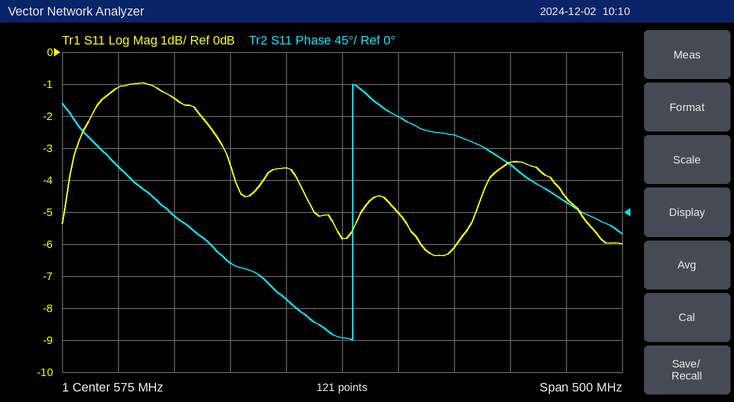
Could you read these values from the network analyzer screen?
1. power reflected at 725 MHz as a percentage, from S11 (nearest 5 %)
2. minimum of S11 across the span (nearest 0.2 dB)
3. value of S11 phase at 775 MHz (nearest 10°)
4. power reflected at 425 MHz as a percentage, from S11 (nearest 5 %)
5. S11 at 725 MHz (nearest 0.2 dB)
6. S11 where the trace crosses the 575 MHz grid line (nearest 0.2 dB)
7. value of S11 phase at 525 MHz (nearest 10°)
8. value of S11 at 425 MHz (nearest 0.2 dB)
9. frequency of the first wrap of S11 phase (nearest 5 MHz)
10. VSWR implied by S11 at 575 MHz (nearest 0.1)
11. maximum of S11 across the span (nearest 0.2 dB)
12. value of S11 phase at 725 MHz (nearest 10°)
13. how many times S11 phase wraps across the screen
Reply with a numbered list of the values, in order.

1. 45 %
2. -6.4 dB
3. 10°
4. 70 %
5. -3.4 dB
6. -5.8 dB
7. -120°
8. -1.4 dB
9. 585 MHz
10. 3.1
11. -1.0 dB
12. 70°
13. 1
